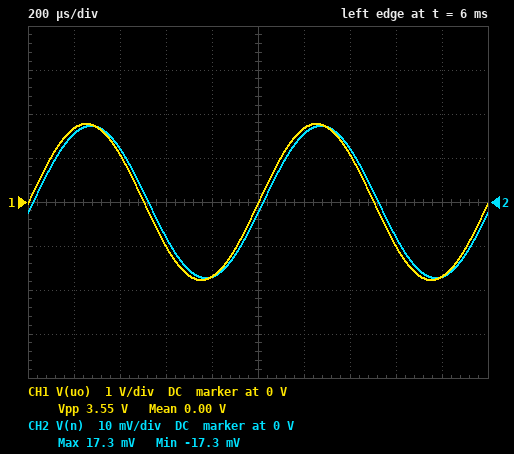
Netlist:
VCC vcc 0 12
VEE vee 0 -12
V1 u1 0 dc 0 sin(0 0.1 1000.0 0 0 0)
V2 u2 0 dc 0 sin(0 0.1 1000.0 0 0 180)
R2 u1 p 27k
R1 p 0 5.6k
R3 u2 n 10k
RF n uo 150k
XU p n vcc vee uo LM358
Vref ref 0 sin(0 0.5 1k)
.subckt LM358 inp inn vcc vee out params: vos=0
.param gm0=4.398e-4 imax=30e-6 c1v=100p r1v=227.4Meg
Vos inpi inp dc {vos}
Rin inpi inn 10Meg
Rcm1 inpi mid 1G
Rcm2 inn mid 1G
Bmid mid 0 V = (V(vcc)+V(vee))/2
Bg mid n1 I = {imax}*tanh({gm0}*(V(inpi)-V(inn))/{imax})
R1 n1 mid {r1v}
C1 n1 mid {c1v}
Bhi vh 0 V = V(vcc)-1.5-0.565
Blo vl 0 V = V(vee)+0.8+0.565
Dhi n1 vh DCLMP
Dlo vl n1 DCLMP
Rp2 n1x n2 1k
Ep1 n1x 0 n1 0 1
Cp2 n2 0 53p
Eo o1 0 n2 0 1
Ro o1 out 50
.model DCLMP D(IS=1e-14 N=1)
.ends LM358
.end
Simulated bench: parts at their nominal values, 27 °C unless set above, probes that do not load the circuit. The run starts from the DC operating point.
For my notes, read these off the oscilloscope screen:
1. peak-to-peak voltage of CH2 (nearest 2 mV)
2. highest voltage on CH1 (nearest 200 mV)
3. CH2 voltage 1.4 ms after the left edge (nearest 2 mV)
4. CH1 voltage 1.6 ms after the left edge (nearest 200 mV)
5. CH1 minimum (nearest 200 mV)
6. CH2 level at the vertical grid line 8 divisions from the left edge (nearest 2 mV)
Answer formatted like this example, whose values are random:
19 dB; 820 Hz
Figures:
34 mV; 1.8 V; 12 mV; -1.0 V; -1.8 V; -8 mV
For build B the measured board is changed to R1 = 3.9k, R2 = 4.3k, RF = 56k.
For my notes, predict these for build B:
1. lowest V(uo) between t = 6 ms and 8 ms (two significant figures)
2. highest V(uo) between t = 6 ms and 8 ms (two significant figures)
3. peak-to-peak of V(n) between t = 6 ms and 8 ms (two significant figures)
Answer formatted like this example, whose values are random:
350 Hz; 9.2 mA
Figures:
-870 mV; 870 mV; 95 mV
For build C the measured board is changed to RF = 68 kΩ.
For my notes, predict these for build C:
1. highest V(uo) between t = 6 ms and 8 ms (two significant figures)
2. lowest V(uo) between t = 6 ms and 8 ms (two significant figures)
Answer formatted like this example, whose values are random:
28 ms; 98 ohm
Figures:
810 mV; -810 mV
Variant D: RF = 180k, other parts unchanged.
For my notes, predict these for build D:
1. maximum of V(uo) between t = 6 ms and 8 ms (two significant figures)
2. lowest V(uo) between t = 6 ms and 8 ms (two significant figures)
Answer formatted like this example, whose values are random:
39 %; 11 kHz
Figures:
2.1 V; -2.1 V
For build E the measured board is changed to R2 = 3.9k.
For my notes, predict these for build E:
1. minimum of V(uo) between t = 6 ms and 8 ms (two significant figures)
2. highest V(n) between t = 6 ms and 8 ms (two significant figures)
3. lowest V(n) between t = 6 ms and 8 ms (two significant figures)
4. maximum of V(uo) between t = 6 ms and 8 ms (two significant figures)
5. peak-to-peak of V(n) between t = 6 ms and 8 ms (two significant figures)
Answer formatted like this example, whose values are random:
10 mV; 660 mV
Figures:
-2.4 V; 59 mV; -59 mV; 2.4 V; 120 mV
